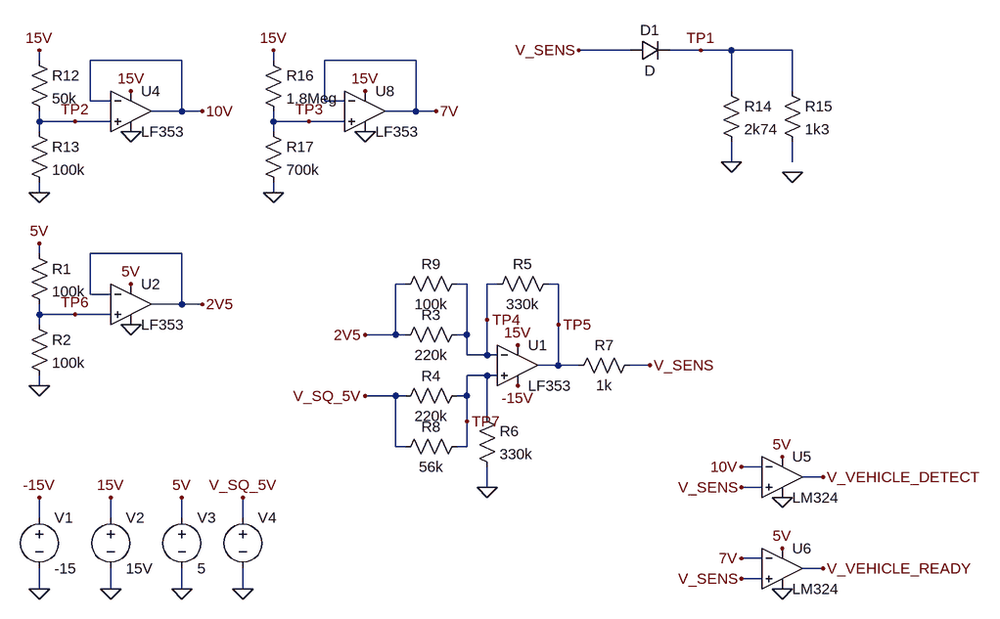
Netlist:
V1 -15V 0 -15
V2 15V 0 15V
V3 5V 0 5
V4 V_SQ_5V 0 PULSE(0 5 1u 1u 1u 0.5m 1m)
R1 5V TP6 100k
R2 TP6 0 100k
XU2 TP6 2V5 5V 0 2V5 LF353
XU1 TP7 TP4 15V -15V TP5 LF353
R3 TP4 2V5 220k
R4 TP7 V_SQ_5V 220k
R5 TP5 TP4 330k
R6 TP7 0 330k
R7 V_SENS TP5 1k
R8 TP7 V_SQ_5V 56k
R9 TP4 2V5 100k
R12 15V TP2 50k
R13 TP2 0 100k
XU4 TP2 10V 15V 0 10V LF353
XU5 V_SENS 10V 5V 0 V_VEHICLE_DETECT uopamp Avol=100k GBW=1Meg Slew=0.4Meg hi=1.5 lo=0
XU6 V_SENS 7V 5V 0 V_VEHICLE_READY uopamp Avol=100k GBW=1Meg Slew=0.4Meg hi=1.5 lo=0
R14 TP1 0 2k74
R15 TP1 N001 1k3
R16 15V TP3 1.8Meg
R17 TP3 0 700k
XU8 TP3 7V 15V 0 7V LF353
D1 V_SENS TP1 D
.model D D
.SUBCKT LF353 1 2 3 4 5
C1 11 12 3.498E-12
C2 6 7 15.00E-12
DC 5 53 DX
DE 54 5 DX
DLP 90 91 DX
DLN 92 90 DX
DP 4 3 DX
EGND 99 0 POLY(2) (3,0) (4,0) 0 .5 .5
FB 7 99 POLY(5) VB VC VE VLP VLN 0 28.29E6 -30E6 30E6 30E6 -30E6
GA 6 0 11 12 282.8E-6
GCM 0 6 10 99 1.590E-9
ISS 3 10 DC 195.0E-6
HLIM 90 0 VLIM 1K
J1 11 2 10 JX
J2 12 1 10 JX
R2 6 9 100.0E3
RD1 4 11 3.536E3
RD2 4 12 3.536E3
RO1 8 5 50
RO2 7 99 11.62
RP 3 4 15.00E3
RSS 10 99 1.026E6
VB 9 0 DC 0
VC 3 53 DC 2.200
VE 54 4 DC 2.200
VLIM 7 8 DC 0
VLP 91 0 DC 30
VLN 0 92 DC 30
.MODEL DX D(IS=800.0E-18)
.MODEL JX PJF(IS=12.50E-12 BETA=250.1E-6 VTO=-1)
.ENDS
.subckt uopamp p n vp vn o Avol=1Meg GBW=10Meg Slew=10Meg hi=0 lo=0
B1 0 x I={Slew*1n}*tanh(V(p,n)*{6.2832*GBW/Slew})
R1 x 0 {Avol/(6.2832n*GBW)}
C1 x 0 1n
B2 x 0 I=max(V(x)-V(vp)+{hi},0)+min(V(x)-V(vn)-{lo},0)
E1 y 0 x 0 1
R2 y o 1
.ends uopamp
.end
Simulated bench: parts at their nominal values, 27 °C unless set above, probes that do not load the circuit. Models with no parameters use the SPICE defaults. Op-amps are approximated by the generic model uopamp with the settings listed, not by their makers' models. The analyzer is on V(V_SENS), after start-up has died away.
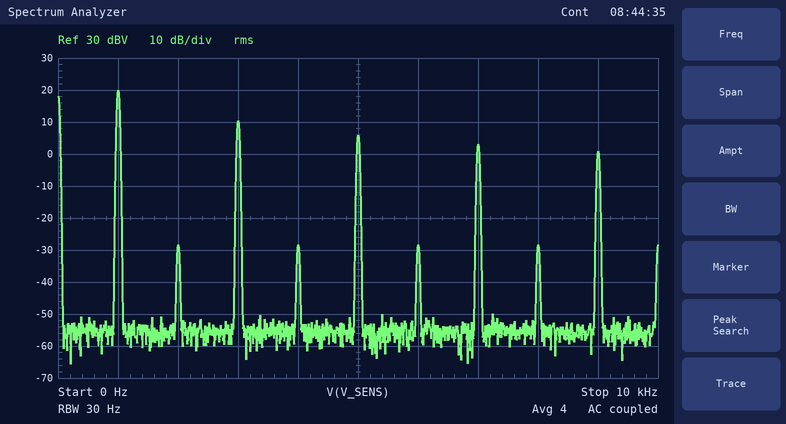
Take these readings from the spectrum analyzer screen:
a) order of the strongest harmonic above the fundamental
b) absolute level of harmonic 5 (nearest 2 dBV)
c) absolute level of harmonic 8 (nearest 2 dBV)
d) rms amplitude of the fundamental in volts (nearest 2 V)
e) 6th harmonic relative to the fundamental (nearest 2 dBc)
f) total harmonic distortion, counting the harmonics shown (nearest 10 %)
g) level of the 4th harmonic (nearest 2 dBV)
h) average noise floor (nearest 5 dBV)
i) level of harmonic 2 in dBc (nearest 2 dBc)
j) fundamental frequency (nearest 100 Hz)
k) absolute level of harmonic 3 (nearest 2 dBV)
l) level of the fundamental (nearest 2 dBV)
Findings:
3
6 dBV
-28 dBV
10 V
-48 dBc
40 %
-28 dBV
-55 dBV
-48 dBc
1.0 kHz
10 dBV
20 dBV
